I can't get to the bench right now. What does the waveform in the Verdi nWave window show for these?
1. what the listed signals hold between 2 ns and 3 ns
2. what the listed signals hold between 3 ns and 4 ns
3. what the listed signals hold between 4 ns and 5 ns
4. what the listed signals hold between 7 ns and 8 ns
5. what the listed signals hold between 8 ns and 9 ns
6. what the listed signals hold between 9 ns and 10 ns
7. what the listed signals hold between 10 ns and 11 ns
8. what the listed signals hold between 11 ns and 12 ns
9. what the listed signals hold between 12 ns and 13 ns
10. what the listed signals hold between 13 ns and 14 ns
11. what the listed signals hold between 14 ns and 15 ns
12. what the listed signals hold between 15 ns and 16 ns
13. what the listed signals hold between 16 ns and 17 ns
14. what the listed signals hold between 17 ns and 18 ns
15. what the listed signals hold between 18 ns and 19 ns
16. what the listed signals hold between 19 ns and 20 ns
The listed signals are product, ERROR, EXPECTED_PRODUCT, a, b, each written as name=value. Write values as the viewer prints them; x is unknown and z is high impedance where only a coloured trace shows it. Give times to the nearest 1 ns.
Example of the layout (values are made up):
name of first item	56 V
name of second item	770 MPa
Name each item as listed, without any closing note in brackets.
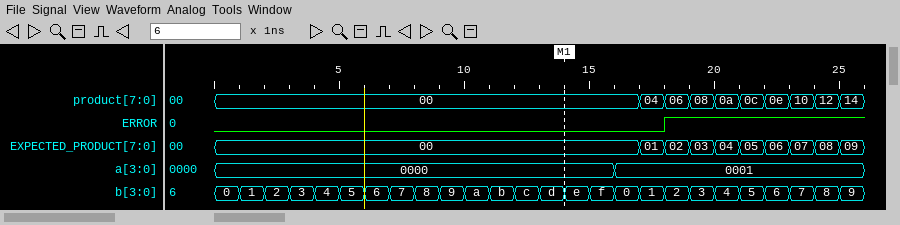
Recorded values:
what the listed signals hold between 2 ns and 3 ns	product=00, ERROR=0, EXPECTED_PRODUCT=00, a=0000, b=2
what the listed signals hold between 3 ns and 4 ns	product=00, ERROR=0, EXPECTED_PRODUCT=00, a=0000, b=3
what the listed signals hold between 4 ns and 5 ns	product=00, ERROR=0, EXPECTED_PRODUCT=00, a=0000, b=4
what the listed signals hold between 7 ns and 8 ns	product=00, ERROR=0, EXPECTED_PRODUCT=00, a=0000, b=7
what the listed signals hold between 8 ns and 9 ns	product=00, ERROR=0, EXPECTED_PRODUCT=00, a=0000, b=8
what the listed signals hold between 9 ns and 10 ns	product=00, ERROR=0, EXPECTED_PRODUCT=00, a=0000, b=9
what the listed signals hold between 10 ns and 11 ns	product=00, ERROR=0, EXPECTED_PRODUCT=00, a=0000, b=a
what the listed signals hold between 11 ns and 12 ns	product=00, ERROR=0, EXPECTED_PRODUCT=00, a=0000, b=b
what the listed signals hold between 12 ns and 13 ns	product=00, ERROR=0, EXPECTED_PRODUCT=00, a=0000, b=c
what the listed signals hold between 13 ns and 14 ns	product=00, ERROR=0, EXPECTED_PRODUCT=00, a=0000, b=d
what the listed signals hold between 14 ns and 15 ns	product=00, ERROR=0, EXPECTED_PRODUCT=00, a=0000, b=e
what the listed signals hold between 15 ns and 16 ns	product=00, ERROR=0, EXPECTED_PRODUCT=00, a=0000, b=f
what the listed signals hold between 16 ns and 17 ns	product=00, ERROR=0, EXPECTED_PRODUCT=00, a=0001, b=0
what the listed signals hold between 17 ns and 18 ns	product=04, ERROR=0, EXPECTED_PRODUCT=01, a=0001, b=1
what the listed signals hold between 18 ns and 19 ns	product=06, ERROR=1, EXPECTED_PRODUCT=02, a=0001, b=2
what the listed signals hold between 19 ns and 20 ns	product=08, ERROR=1, EXPECTED_PRODUCT=03, a=0001, b=3
